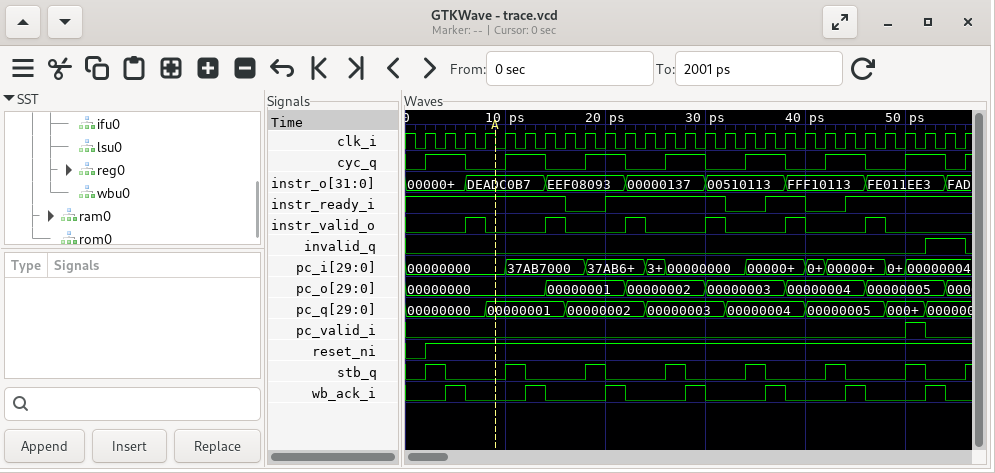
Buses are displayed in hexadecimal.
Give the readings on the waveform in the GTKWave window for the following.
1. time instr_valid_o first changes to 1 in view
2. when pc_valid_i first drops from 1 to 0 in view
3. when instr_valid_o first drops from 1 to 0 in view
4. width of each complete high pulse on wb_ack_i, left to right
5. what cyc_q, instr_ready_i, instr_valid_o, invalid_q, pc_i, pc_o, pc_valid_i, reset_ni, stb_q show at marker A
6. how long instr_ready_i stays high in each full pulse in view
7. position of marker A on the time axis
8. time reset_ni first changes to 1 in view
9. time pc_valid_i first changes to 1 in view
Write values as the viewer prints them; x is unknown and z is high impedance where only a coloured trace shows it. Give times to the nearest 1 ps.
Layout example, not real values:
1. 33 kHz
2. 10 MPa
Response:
1. 6 ps
2. 52 ps
3. 8 ps
4. 2 ps, 2 ps, 2 ps, 2 ps, 2 ps, 2 ps, 2 ps
5. cyc_q=0, instr_ready_i=1, instr_valid_o=0, invalid_q=0, pc_i=00000000, pc_o=00000000, pc_valid_i=0, reset_ni=1, stb_q=0
6. 12 ps, 4 ps
7. 9 ps
8. 2 ps
9. 50 ps
